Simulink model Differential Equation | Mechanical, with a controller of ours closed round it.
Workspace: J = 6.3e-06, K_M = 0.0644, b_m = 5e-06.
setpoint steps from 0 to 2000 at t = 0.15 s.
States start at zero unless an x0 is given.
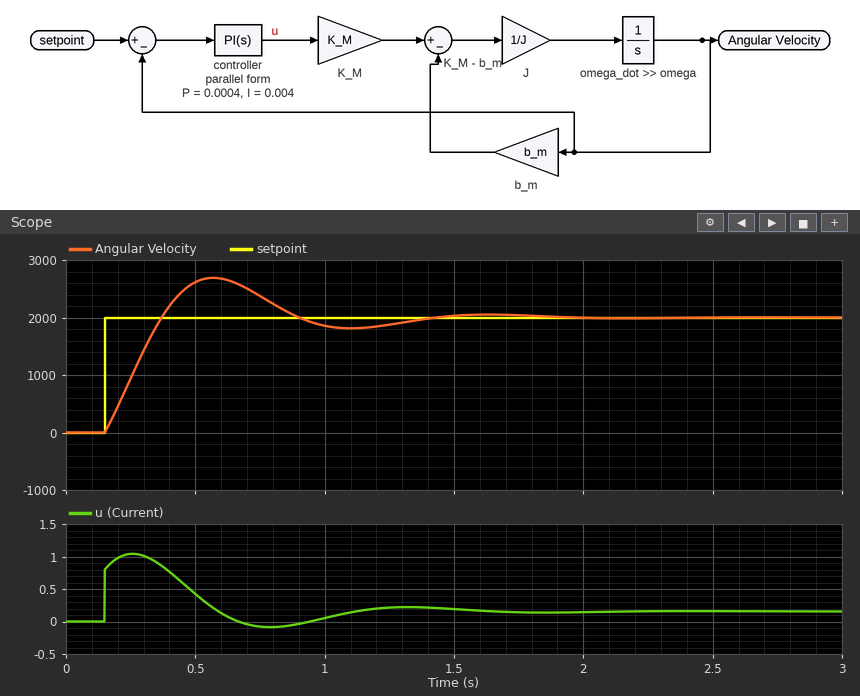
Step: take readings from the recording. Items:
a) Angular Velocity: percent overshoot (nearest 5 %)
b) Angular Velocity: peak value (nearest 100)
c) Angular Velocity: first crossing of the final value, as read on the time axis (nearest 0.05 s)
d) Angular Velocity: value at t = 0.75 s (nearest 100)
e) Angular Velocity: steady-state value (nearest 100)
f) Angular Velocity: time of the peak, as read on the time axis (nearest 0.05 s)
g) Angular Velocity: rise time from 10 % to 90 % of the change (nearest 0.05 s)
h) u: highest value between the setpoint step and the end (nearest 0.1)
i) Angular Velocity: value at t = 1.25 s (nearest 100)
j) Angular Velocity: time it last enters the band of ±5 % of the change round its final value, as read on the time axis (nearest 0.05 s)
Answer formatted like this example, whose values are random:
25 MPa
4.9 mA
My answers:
35 %
2700
0.35 s
2400
2000
0.55 s
0.15 s
1.0
1900
1.30 s
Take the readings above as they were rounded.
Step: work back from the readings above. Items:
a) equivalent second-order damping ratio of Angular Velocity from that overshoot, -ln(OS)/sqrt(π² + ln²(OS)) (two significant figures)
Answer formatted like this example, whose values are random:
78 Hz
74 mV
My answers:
0.32
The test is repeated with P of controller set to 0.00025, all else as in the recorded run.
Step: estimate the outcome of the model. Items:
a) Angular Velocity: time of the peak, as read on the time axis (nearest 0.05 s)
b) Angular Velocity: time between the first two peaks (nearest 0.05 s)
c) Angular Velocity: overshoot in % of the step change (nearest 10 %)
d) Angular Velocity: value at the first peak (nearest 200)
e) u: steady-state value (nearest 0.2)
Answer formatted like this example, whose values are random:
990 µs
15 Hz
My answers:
0.60 s
1.00 s
50 %
3000
0.2
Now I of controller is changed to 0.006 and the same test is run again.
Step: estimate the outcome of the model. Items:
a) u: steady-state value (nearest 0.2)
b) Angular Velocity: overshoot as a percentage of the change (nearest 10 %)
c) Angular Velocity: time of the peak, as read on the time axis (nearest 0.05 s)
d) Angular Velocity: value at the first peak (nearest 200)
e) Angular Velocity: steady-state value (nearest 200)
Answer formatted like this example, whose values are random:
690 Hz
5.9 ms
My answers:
0.2
40 %
0.50 s
2800
2000
